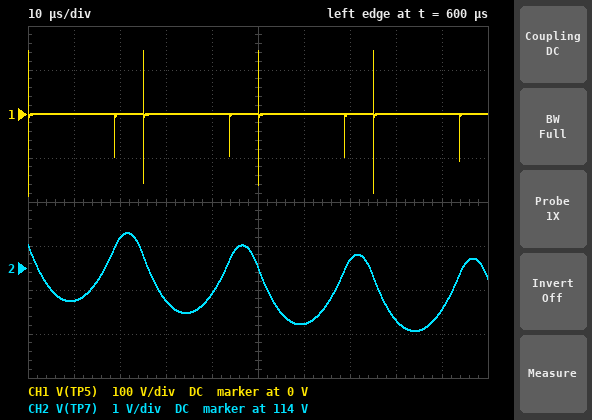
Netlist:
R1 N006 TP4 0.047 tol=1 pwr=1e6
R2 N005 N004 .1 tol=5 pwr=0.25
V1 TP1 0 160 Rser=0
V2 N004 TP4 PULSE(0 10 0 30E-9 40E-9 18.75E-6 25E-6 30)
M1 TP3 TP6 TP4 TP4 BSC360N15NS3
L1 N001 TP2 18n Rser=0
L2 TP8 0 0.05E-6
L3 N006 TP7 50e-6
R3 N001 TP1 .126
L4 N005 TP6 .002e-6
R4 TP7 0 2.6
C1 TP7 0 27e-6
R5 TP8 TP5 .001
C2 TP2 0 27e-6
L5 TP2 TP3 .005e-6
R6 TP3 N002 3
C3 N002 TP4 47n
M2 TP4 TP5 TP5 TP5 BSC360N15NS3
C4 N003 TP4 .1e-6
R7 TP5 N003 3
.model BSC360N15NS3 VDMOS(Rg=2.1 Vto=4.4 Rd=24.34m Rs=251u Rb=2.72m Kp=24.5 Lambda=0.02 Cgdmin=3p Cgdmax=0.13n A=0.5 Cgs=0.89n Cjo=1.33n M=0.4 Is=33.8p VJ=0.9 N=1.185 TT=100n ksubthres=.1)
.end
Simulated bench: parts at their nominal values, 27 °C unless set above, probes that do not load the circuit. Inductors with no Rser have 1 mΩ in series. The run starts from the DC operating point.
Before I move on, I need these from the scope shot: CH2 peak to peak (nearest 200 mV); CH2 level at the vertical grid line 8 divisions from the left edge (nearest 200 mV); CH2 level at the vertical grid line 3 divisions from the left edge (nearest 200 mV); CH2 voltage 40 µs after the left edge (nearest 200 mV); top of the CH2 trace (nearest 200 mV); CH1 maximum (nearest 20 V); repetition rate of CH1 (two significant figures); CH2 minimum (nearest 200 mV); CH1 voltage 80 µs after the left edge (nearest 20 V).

2.2 V
112.8 V
113.2 V
113.4 V
114.8 V
140 V
40 kHz
112.6 V
0 V
